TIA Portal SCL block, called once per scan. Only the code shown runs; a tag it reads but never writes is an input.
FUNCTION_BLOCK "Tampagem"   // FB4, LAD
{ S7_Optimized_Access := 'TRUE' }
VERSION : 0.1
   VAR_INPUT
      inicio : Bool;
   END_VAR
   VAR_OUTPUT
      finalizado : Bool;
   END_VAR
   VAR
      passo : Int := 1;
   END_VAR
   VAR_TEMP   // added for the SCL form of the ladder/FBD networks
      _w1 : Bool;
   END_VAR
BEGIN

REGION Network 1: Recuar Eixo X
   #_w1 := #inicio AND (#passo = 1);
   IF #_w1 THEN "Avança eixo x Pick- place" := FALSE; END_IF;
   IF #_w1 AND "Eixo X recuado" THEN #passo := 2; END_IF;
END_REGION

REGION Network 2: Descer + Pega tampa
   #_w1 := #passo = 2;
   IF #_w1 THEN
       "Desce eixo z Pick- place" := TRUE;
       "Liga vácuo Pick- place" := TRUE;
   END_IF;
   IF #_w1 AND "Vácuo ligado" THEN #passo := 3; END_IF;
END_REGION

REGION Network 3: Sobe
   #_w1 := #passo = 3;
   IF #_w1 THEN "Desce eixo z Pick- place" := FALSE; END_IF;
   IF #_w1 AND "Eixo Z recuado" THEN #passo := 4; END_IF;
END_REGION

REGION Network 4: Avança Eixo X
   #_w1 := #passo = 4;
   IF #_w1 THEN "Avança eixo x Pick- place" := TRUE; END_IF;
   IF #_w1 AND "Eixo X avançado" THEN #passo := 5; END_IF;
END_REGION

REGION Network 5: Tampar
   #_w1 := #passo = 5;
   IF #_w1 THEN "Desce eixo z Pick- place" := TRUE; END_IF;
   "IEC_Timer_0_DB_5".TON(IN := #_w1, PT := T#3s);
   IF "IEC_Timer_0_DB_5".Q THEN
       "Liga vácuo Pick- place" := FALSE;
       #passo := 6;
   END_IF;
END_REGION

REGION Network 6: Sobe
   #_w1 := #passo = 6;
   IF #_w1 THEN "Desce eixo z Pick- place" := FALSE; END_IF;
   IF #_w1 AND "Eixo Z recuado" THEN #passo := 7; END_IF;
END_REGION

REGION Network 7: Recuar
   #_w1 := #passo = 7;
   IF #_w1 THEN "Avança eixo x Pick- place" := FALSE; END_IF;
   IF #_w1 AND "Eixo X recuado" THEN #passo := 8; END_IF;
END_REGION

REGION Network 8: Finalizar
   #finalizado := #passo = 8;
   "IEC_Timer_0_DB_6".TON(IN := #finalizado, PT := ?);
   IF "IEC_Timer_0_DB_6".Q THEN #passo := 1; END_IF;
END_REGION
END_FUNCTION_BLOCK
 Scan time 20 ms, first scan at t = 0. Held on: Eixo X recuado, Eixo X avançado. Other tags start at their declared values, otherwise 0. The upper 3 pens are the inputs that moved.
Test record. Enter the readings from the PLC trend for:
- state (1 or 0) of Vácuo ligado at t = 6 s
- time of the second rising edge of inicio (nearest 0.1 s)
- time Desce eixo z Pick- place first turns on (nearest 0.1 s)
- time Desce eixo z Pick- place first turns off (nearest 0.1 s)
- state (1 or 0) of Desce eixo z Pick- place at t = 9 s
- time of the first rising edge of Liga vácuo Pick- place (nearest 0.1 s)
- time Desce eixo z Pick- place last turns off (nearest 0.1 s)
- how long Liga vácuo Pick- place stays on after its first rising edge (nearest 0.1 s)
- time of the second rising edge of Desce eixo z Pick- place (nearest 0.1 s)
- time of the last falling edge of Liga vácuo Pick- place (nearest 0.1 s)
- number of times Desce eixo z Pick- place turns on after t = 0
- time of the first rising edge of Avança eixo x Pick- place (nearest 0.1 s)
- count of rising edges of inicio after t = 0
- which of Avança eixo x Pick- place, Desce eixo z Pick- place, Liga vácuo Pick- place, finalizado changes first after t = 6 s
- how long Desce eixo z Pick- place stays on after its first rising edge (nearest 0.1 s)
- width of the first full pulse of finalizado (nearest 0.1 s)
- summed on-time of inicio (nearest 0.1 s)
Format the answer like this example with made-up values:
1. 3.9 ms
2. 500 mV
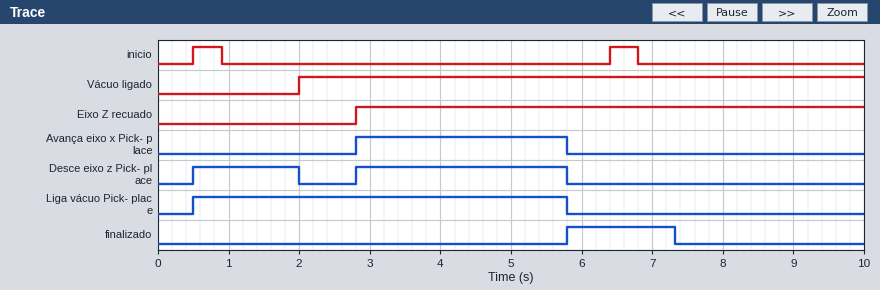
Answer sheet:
1. 1
2. 6.4 s
3. 0.5 s
4. 2.0 s
5. 0
6. 0.5 s
7. 5.8 s
8. 5.3 s
9. 2.8 s
10. 5.8 s
11. 2
12. 2.8 s
13. 2
14. finalizado
15. 1.5 s
16. 1.5 s
17. 0.8 s
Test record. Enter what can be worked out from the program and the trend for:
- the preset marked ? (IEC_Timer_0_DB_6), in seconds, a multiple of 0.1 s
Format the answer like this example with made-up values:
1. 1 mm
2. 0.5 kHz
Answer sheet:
1. 1.5 s
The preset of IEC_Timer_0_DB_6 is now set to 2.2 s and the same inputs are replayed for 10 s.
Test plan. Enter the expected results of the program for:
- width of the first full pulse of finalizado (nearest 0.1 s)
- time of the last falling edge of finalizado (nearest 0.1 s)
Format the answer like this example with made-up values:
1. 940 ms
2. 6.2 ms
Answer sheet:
1. 2.2 s
2. 8.0 s
